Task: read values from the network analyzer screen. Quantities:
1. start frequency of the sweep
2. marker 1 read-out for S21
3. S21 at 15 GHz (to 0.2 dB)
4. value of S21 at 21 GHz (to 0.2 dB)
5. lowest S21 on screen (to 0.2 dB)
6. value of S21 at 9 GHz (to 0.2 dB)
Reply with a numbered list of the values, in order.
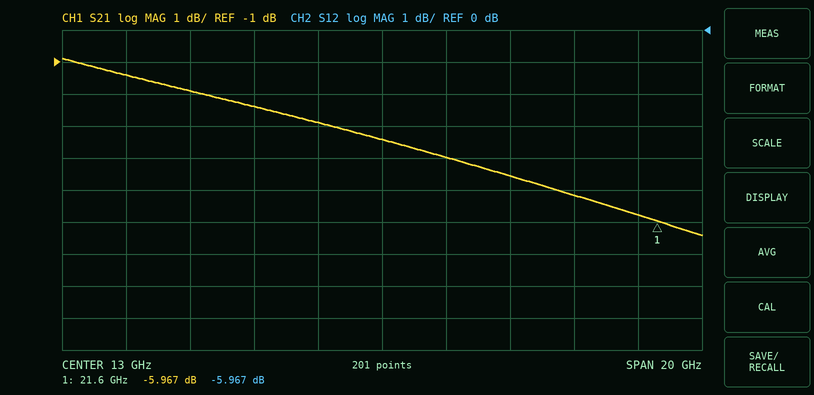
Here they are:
1. 3 GHz
2. -5.967 dB
3. -4.0 dB
4. -5.8 dB
5. -6.4 dB
6. -2.4 dB
